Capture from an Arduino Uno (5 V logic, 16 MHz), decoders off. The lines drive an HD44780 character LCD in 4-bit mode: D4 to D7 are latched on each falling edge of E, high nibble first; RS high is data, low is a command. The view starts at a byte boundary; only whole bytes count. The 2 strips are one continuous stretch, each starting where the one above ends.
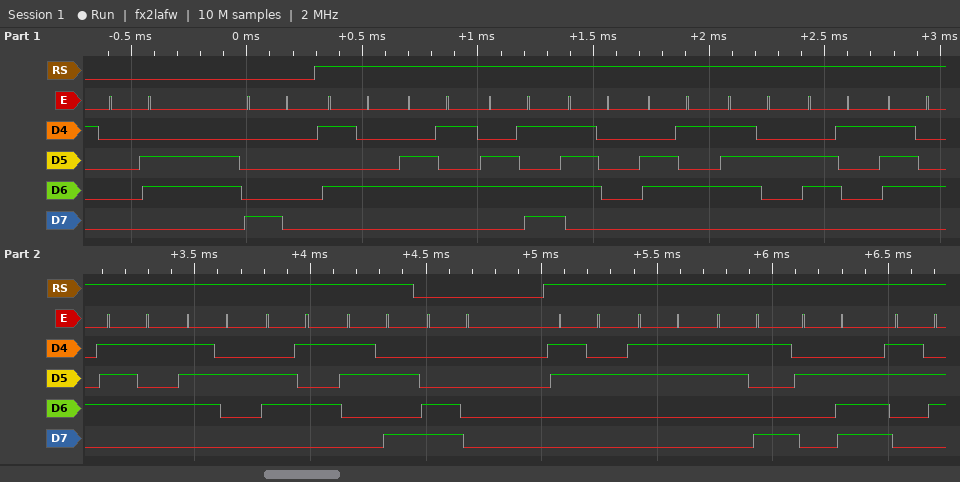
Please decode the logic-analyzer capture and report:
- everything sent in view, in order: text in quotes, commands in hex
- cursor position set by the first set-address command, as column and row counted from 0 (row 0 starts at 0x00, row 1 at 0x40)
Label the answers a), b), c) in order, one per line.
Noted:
a) 0x06 0x80 "Temperature:" 0xC0 "239.6"
b) column 0, row 0
